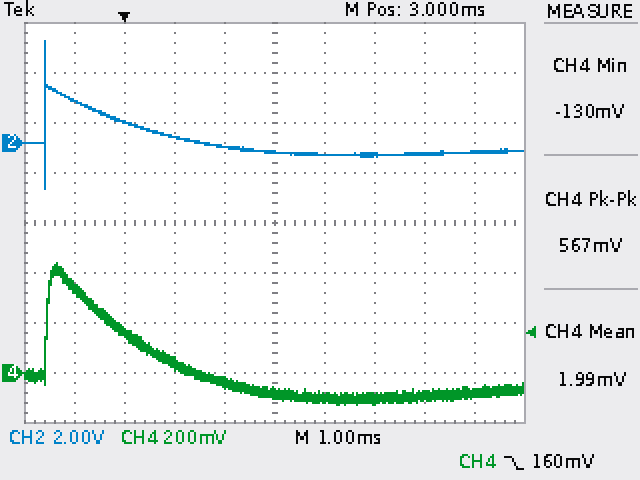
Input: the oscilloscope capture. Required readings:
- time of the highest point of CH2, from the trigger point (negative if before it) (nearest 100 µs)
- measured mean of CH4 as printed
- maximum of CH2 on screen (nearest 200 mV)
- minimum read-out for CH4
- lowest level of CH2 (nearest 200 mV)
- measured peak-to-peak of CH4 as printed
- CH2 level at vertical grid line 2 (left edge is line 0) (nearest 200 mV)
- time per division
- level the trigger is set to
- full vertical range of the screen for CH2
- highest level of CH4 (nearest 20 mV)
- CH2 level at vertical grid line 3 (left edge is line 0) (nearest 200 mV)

-1.6 ms
1.99 mV
4.0 V
-130 mV
-1.8 V
567 mV
800 mV
1 ms
160 mV
16 V
440 mV
200 mV
